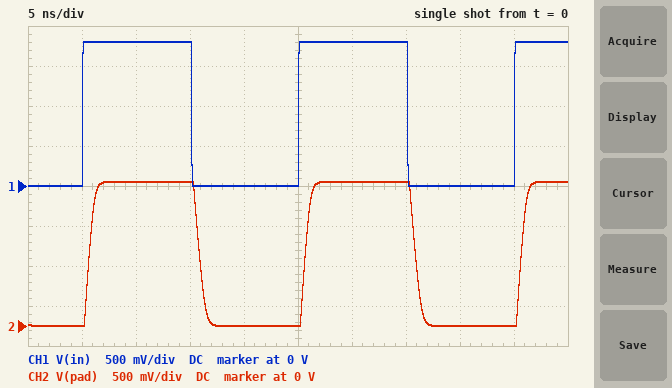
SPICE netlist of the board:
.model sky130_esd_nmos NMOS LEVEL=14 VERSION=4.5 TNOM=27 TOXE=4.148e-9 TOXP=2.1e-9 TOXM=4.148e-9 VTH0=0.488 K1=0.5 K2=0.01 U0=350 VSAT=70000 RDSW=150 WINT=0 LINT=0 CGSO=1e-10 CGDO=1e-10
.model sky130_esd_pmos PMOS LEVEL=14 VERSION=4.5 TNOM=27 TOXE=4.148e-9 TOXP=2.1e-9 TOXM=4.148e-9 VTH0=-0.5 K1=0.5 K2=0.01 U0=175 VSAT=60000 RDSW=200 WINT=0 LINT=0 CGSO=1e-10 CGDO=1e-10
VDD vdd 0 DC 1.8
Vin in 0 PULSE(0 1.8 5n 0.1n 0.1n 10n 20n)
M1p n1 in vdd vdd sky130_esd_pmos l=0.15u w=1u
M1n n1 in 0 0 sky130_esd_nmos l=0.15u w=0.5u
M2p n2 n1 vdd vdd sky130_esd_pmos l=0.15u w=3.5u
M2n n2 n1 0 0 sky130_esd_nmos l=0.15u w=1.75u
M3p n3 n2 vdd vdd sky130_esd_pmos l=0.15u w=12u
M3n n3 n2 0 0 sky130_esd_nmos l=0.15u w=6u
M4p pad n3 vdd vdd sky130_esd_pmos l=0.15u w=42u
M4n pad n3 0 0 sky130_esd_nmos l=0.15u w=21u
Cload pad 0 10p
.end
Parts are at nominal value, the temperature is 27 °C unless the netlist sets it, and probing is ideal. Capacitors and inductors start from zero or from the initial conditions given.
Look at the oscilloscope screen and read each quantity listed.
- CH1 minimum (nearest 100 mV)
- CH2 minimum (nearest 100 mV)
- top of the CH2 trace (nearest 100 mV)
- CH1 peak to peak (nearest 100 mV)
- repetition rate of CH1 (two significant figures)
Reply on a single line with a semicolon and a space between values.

0 V; 0 V; 1.8 V; 1.8 V; 50 MHz
